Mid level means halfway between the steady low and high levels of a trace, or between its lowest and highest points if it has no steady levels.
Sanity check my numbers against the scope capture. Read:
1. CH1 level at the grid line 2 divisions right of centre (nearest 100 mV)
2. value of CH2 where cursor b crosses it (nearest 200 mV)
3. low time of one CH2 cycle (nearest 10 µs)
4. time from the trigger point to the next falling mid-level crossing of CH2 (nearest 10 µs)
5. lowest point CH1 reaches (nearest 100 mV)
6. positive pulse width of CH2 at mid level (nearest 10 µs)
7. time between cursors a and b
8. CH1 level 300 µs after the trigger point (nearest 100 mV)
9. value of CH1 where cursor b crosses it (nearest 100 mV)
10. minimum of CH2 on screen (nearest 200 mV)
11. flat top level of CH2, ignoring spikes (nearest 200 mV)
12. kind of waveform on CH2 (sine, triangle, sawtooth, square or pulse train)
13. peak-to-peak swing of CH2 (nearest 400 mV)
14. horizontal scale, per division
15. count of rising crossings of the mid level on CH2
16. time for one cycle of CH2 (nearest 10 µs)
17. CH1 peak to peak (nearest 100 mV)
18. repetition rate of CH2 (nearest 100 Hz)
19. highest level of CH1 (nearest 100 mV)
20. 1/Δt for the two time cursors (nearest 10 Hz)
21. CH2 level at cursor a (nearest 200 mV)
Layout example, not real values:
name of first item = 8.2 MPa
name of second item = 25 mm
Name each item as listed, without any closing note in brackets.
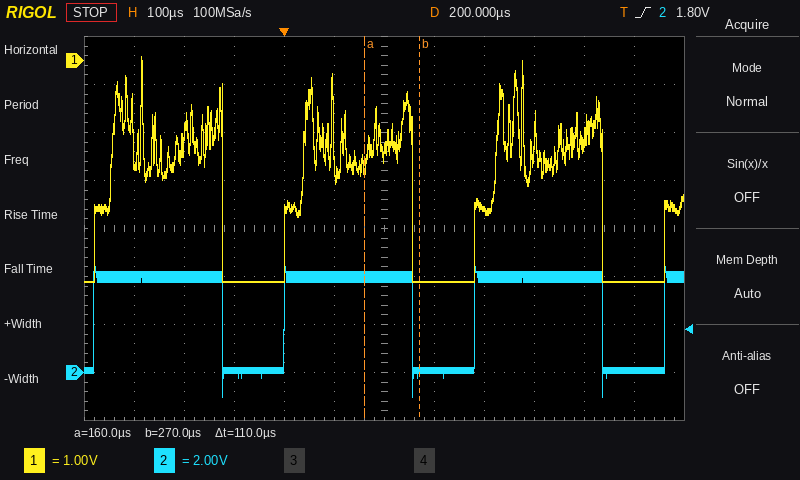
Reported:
CH1 level at the grid line 2 divisions right of centre = -3.1 V
value of CH2 where cursor b crosses it = 0.0 V
low time of one CH2 cycle = 120 µs
time from the trigger point to the next falling mid-level crossing of CH2 = 260 µs
lowest point CH1 reaches = -4.6 V
positive pulse width of CH2 at mid level = 260 µs
time between cursors a and b = 110 µs
CH1 level 300 µs after the trigger point = -4.6 V
value of CH1 where cursor b crosses it = -4.6 V
minimum of CH2 on screen = -1.0 V
flat top level of CH2, ignoring spikes = 4.0 V
kind of waveform on CH2 = pulse train
peak-to-peak swing of CH2 = 5.6 V
horizontal scale, per division = 100 µs
count of rising crossings of the mid level on CH2 = 4
time for one cycle of CH2 = 380 µs
CH1 peak to peak = 4.7 V
repetition rate of CH2 = 2.6 kHz
highest level of CH1 = 100 mV
1/Δt for the two time cursors = 9.09 kHz
CH2 level at cursor a = 4.0 V
